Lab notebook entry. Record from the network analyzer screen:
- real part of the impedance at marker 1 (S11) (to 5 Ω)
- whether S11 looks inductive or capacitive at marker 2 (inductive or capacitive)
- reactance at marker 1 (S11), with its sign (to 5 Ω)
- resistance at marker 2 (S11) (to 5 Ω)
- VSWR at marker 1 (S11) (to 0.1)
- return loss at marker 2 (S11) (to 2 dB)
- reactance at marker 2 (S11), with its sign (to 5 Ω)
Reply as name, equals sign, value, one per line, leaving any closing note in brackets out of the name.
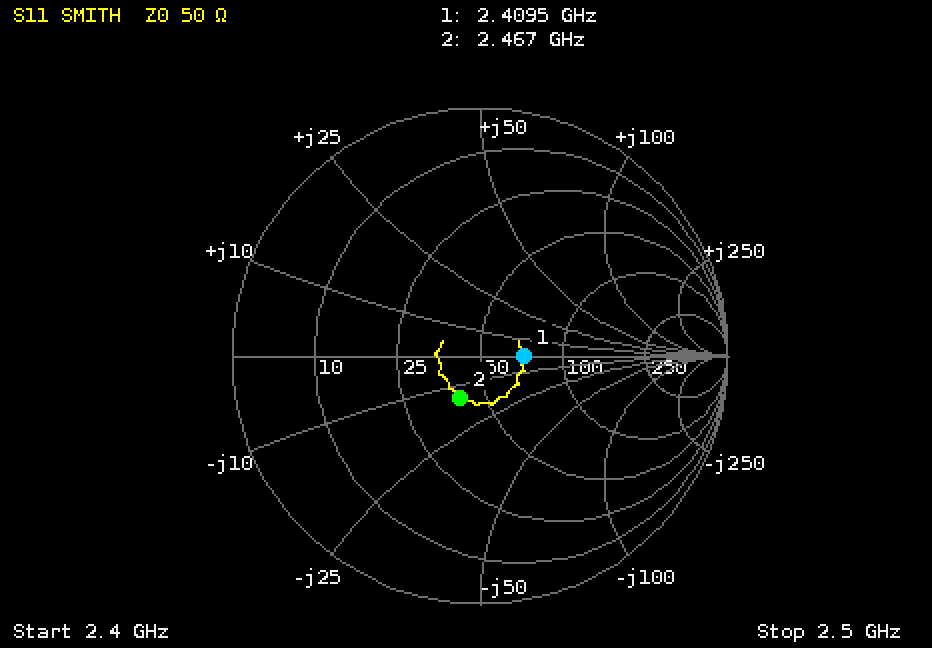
real part of the impedance at marker 1 (S11) = 70 Ω
whether S11 looks inductive or capacitive at marker 2 = capacitive
reactance at marker 1 (S11), with its sign = 0 Ω
resistance at marker 2 (S11) = 40 Ω
VSWR at marker 1 (S11) = 1.4
return loss at marker 2 (S11) = 14 dB
reactance at marker 2 (S11), with its sign = -15 Ω
